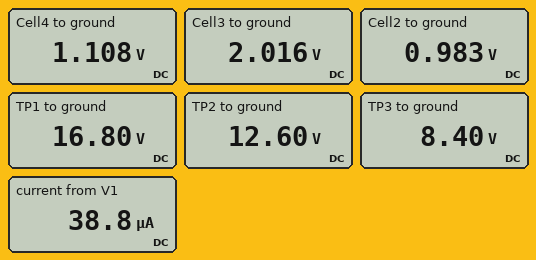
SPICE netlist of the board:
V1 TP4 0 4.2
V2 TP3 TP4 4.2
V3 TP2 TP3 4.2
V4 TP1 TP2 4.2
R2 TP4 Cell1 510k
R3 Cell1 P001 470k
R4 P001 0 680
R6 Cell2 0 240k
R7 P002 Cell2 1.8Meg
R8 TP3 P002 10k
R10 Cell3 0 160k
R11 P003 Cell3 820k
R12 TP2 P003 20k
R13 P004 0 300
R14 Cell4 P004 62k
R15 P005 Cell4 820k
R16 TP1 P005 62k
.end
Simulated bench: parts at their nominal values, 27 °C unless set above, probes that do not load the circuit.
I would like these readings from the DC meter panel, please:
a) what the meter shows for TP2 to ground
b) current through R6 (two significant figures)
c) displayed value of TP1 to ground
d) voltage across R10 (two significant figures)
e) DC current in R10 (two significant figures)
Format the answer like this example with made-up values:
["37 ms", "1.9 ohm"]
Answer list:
["12.60 V", "4.1 µA", "16.80 V", "2.0 V", "13 µA"]
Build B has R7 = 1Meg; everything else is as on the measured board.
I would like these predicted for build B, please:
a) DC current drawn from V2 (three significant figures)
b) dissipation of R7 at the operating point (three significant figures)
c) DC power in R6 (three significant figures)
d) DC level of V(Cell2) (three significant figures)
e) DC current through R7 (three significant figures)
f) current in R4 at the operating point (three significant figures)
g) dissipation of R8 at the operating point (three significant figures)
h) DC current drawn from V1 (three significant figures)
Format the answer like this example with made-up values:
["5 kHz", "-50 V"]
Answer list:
["37.1 µA", "45.2 µW", "10.8 µW", "1.61 V", "6.72 µA", "4.28 µA", "452 nW", "41.4 µA"]
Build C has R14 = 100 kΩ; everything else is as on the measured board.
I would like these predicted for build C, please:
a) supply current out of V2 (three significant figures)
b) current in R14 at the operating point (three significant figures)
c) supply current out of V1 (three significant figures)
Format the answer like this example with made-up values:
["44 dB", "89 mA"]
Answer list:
["33.8 µA", "17.1 µA", "38.1 µA"]
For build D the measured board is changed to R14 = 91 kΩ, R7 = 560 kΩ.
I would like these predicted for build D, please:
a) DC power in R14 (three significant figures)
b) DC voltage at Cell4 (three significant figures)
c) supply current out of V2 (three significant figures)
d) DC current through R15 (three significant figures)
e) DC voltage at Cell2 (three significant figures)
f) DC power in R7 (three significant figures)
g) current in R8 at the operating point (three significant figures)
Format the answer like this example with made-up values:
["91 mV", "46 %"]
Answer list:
["27.1 µW", "1.58 V", "40.2 µA", "17.3 µA", "2.49 V", "60.2 µW", "10.4 µA"]
